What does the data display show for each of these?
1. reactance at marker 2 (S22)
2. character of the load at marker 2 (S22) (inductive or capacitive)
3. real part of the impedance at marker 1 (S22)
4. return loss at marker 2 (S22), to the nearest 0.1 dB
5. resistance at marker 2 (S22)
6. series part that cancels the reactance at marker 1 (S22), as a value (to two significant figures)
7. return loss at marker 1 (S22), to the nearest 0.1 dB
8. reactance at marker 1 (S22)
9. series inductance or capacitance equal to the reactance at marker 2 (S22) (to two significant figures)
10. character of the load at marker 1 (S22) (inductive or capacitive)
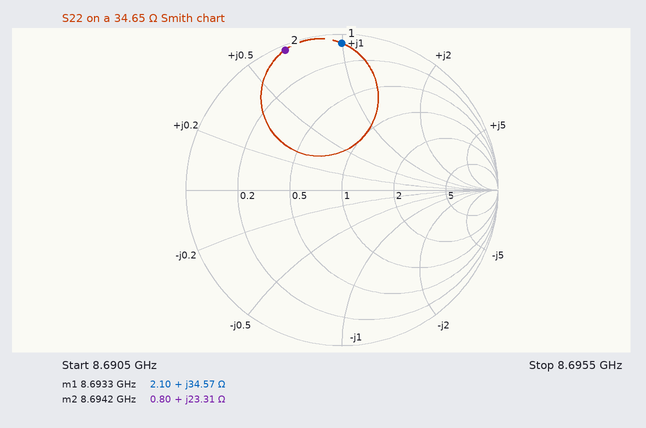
+23.31 Ω
inductive
2.10 Ω
0.3 dB
0.80 Ω
530 fF
0.5 dB
+34.57 Ω
430 pH
inductive
